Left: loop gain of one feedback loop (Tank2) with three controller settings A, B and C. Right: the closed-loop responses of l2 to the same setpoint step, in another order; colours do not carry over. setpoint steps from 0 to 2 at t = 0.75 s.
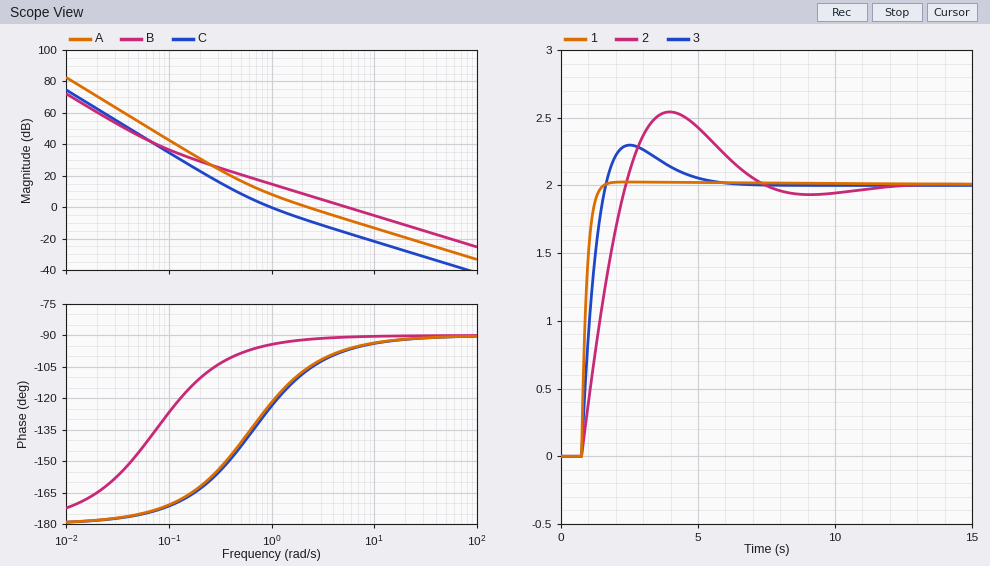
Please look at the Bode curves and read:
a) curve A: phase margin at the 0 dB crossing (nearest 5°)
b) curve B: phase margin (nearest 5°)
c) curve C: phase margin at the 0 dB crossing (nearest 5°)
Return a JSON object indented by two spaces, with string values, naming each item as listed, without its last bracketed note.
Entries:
{
  "curve A: phase margin at the 0 dB crossing": "75°",
  "curve B: phase margin": "90°",
  "curve C: phase margin at the 0 dB crossing": "55°"
}
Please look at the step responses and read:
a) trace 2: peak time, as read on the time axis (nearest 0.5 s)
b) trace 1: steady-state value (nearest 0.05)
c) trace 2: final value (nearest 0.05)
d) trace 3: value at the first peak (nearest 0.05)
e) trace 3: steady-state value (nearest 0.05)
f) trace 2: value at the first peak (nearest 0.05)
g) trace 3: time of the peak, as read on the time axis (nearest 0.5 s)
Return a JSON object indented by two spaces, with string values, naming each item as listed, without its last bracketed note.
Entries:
{
  "trace 2: peak time, as read on the time axis": "4.0 s",
  "trace 1: steady-state value": "2.00",
  "trace 2: final value": "2.00",
  "trace 3: value at the first peak": "2.30",
  "trace 3: steady-state value": "2.00",
  "trace 2: value at the first peak": "2.55",
  "trace 3: time of the peak, as read on the time axis": "2.5 s"
}
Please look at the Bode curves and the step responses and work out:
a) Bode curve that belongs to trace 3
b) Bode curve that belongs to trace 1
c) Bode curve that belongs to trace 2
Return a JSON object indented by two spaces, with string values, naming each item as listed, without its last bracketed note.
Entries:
{
  "Bode curve that belongs to trace 3": "A",
  "Bode curve that belongs to trace 1": "B",
  "Bode curve that belongs to trace 2": "C"
}
